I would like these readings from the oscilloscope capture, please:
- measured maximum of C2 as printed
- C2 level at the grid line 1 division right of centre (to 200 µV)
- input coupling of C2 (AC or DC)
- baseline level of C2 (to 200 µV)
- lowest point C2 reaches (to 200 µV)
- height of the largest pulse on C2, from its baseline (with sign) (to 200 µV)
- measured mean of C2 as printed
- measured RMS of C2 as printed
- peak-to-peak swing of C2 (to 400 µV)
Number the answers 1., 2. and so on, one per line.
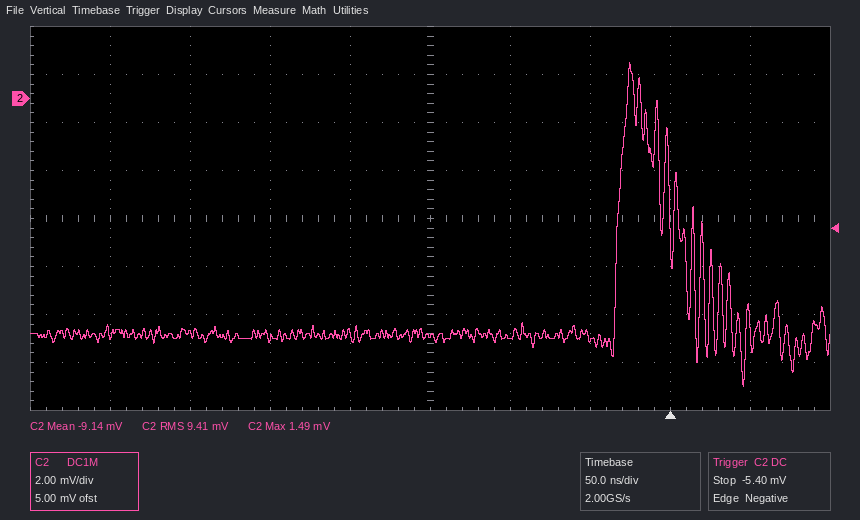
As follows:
1. 1.49 mV
2. -9.8 mV
3. DC
4. -9.8 mV
5. -12.0 mV
6. +11.4 mV
7. -9.14 mV
8. 9.41 mV
9. 13.6 mV
